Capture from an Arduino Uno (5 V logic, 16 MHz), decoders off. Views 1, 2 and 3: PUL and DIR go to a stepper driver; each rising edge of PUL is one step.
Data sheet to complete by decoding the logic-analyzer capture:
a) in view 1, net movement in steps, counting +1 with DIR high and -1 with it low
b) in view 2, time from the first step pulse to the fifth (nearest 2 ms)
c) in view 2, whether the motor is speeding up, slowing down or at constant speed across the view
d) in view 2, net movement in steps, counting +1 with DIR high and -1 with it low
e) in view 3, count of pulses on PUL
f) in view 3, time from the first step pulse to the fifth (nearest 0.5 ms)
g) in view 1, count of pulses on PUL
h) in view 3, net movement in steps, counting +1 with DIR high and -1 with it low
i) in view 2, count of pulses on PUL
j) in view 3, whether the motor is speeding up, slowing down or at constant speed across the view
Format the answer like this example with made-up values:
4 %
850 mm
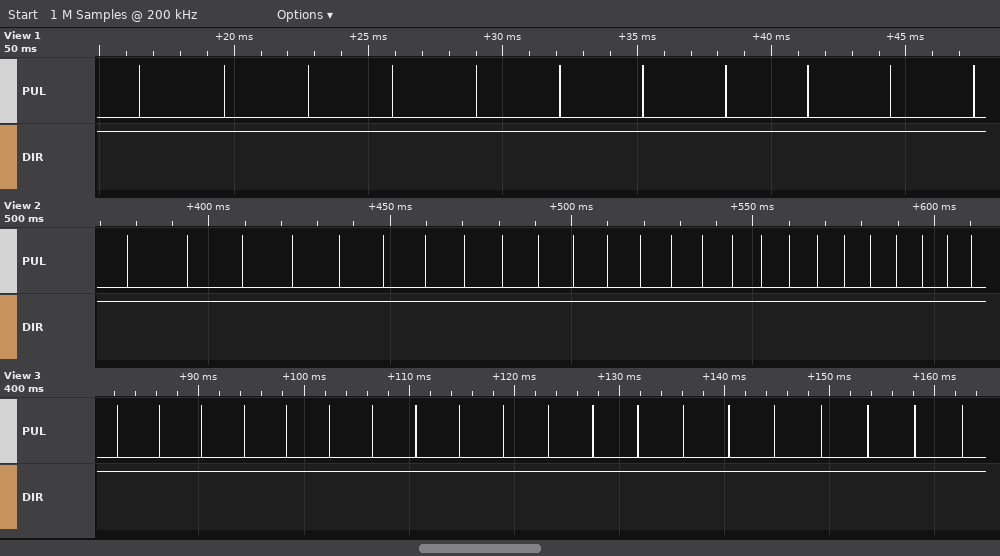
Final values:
+11
58 ms
speeding up
+25
20
16.0 ms
11
+20
25
slowing down
